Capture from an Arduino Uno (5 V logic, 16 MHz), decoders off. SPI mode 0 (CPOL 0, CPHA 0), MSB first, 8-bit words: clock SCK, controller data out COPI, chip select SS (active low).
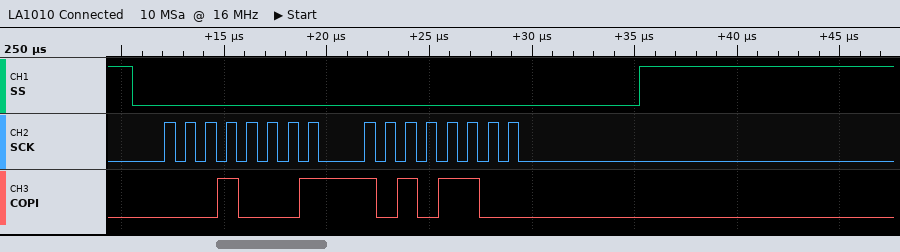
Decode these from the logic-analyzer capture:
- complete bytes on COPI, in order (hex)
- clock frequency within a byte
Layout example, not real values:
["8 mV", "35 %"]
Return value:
["11 AC", "1 MHz"]
